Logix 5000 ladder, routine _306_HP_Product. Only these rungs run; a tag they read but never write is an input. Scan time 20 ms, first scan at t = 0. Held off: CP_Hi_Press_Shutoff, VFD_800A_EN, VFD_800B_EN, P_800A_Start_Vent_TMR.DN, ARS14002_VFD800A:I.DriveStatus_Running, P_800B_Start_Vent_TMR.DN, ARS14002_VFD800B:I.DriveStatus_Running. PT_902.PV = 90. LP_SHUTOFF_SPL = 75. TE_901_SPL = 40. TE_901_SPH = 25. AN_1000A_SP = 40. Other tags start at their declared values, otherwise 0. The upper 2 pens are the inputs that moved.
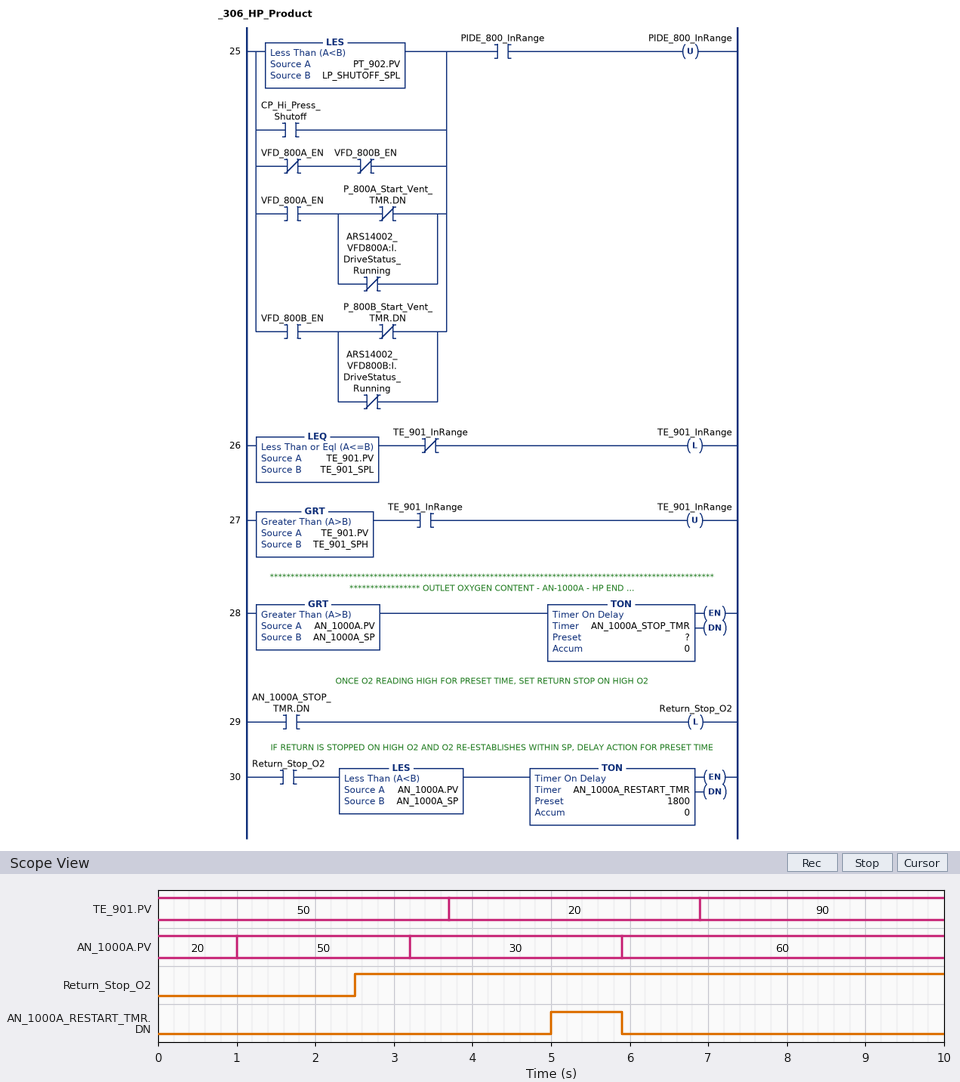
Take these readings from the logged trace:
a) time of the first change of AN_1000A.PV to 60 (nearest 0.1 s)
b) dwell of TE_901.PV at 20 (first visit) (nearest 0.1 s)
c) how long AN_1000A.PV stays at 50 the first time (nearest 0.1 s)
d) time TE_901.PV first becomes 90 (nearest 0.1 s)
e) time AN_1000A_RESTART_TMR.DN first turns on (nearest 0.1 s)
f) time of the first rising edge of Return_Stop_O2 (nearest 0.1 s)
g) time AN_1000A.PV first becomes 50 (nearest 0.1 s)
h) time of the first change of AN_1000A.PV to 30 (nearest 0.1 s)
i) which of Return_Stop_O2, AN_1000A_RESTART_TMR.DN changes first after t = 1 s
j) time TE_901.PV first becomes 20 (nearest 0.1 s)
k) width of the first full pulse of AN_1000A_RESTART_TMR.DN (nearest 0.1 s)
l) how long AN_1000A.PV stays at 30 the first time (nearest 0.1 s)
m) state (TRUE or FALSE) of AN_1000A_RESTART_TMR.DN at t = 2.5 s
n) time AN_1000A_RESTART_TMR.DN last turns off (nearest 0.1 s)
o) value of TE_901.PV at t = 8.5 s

5.9 s
3.2 s
2.2 s
6.9 s
5.0 s
2.5 s
1.0 s
3.2 s
Return_Stop_O2
3.7 s
0.9 s
2.7 s
FALSE
5.9 s
90
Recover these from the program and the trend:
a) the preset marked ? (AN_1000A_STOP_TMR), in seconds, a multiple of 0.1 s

1.5 s
